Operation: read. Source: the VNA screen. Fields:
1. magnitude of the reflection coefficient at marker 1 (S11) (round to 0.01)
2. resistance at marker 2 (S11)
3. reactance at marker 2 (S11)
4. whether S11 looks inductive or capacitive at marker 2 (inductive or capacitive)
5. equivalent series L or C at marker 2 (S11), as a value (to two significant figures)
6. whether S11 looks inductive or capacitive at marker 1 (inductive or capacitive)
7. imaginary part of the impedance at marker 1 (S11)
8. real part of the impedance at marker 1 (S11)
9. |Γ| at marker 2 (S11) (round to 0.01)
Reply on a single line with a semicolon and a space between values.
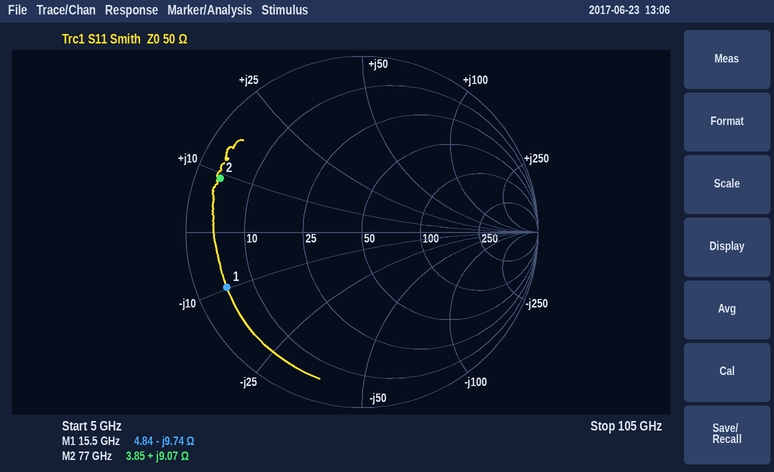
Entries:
0.83; 3.85 Ω; +9.07 Ω; inductive; 19 pH; capacitive; -9.74 Ω; 4.84 Ω; 0.86
